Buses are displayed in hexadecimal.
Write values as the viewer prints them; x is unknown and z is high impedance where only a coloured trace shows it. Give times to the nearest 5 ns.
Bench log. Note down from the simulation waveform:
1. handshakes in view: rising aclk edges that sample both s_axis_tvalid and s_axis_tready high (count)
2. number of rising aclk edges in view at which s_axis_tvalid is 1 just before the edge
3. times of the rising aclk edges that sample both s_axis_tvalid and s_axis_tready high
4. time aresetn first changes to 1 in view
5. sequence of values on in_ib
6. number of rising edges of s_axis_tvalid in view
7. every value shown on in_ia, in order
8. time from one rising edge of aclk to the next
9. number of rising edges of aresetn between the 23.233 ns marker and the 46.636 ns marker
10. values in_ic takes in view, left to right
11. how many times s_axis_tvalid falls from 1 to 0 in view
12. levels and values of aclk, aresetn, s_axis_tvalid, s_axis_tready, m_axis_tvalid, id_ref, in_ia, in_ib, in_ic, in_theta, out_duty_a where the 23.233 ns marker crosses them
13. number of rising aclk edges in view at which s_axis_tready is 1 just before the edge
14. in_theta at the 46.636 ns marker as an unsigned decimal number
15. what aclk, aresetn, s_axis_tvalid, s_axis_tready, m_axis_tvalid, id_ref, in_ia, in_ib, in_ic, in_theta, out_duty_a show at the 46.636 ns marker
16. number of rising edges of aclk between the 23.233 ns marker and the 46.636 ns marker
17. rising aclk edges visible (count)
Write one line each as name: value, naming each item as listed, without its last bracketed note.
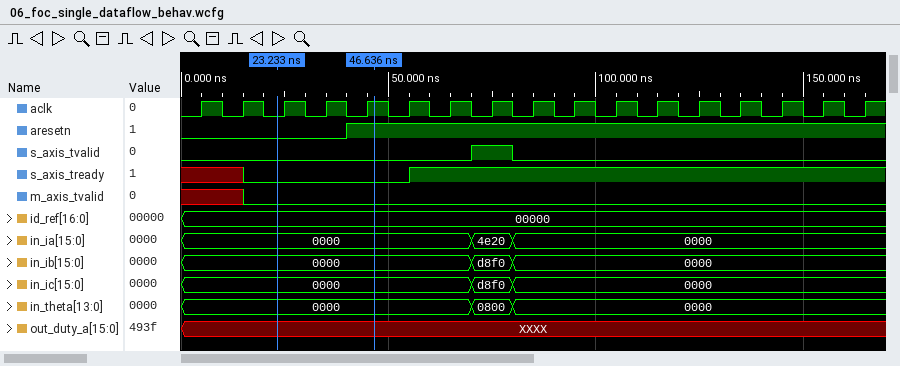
handshakes in view: rising aclk edges that sample both s_axis_tvalid and s_axis_tready high: 1
number of rising aclk edges in view at which s_axis_tvalid is 1 just before the edge: 1
times of the rising aclk edges that sample both s_axis_tvalid and s_axis_tready high: 75 ns
time aresetn first changes to 1 in view: 40 ns
sequence of values on in_ib: 0000, d8f0, 0000
number of rising edges of s_axis_tvalid in view: 1
every value shown on in_ia, in order: 0000, 4e20, 0000
time from one rising edge of aclk to the next: 10 ns
number of rising edges of aresetn between the 23.233 ns marker and the 46.636 ns marker: 1
values in_ic takes in view, left to right: 0000, d8f0, 0000
how many times s_axis_tvalid falls from 1 to 0 in view: 1
levels and values of aclk, aresetn, s_axis_tvalid, s_axis_tready, m_axis_tvalid, id_ref, in_ia, in_ib, in_ic, in_theta, out_duty_a where the 23.233 ns marker crosses them: aclk=0, aresetn=0, s_axis_tvalid=0, s_axis_tready=0, m_axis_tvalid=0, id_ref=00000, in_ia=0000, in_ib=0000, in_ic=0000, in_theta=0000, out_duty_a=XXXX
number of rising aclk edges in view at which s_axis_tready is 1 just before the edge: 11
in_theta at the 46.636 ns marker as an unsigned decimal number: 0
what aclk, aresetn, s_axis_tvalid, s_axis_tready, m_axis_tvalid, id_ref, in_ia, in_ib, in_ic, in_theta, out_duty_a show at the 46.636 ns marker: aclk=1, aresetn=1, s_axis_tvalid=0, s_axis_tready=0, m_axis_tvalid=0, id_ref=00000, in_ia=0000, in_ib=0000, in_ic=0000, in_theta=0000, out_duty_a=XXXX
number of rising edges of aclk between the 23.233 ns marker and the 46.636 ns marker: 3
rising aclk edges visible: 17
